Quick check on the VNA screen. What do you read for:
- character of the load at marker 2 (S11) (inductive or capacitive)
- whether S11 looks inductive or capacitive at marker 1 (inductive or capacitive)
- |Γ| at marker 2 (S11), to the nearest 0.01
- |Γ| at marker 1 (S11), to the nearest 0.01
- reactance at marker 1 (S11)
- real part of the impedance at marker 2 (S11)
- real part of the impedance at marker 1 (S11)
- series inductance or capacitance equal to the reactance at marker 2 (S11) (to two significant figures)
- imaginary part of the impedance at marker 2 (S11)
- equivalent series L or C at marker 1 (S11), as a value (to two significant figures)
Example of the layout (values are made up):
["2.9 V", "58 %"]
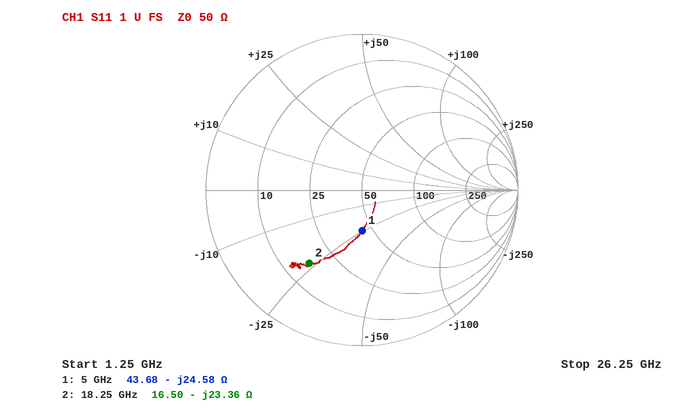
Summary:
["capacitive", "capacitive", "0.58", "0.26", "-24.58 Ω", "16.50 Ω", "43.68 Ω", "370 fF", "-23.36 Ω", "1.3 pF"]
